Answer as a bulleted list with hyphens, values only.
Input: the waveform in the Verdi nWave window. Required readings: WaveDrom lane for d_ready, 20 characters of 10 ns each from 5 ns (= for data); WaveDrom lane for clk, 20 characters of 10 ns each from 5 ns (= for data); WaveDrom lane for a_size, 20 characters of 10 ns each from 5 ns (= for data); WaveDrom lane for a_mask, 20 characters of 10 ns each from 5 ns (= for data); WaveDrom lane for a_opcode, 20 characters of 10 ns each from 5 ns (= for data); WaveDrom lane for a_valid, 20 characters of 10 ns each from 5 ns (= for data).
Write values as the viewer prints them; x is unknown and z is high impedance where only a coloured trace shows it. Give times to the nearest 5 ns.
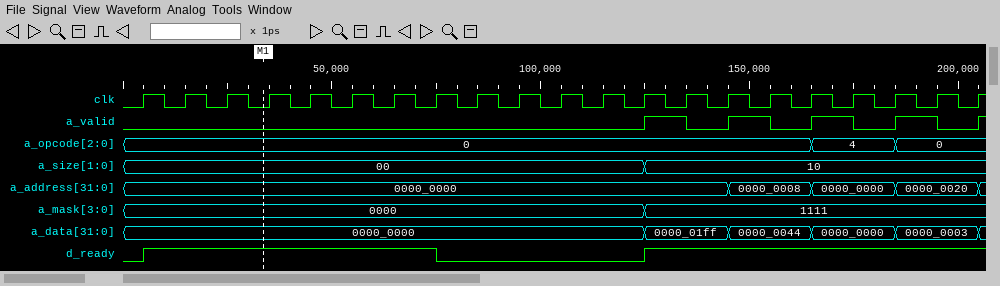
- {name: 'd_ready', wave: '1......0....1.......'}
- {name: 'clk', wave: 'p...................'}
- {name: 'a_size', wave: '=...........=.......', data: '00 10'}
- {name: 'a_mask', wave: '=...........=.......', data: '0000 1111'}
- {name: 'a_opcode', wave: '=...............=.=.', data: '0 4 0'}
- {name: 'a_valid', wave: '0...........10101010'}
